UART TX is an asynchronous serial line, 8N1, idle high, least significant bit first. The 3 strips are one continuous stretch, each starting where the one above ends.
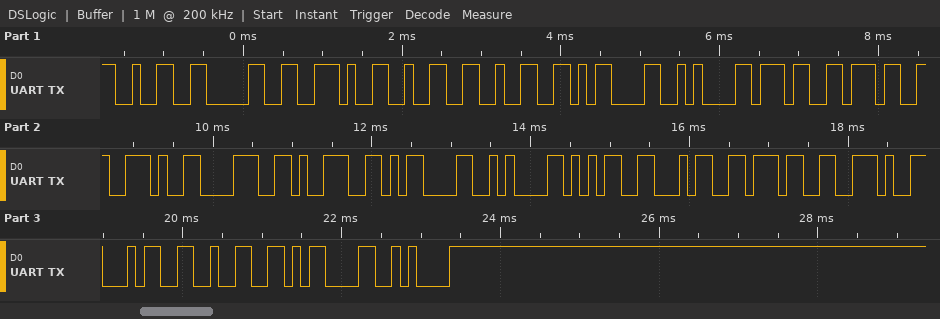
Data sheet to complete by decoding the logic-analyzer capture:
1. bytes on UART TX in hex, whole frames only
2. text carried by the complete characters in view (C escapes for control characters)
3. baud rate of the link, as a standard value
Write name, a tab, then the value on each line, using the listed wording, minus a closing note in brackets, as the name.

bytes on UART TX in hex, whole frames only	0x32 0x30 0x2E 0x32 0x32 0x0D 0x0A 0x37 0x37 0x2E 0x38 0x39 0x0D 0x0A 0x35 0x34 0x37 0x2E 0x34 0x32 0x0D 0x0A
text carried by the complete characters in view	"20.22\r\n77.89\r\n547.42\r\n"
baud rate of the link, as a standard value	9600 baud
